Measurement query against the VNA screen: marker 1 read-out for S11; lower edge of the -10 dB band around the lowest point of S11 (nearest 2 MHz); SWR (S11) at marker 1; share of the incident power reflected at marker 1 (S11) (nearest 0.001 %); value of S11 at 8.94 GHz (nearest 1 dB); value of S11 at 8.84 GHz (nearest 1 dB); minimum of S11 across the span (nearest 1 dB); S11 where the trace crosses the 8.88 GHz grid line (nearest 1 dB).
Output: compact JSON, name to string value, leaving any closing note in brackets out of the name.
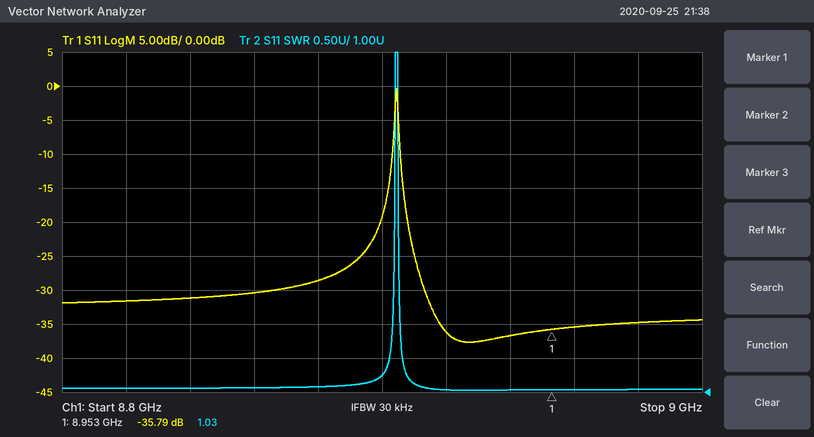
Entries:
{"marker 1 read-out for S11": "-35.79 dB", "lower edge of the -10 dB band around the lowest point of S11": "8.906 GHz", "SWR (S11) at marker 1": "1.03", "share of the incident power reflected at marker 1 (S11)": "0.026 %", "value of S11 at 8.94 GHz": "-37 dB", "value of S11 at 8.84 GHz": "-31 dB", "minimum of S11 across the span": "-38 dB", "S11 where the trace crosses the 8.88 GHz grid line": "-29 dB"}
